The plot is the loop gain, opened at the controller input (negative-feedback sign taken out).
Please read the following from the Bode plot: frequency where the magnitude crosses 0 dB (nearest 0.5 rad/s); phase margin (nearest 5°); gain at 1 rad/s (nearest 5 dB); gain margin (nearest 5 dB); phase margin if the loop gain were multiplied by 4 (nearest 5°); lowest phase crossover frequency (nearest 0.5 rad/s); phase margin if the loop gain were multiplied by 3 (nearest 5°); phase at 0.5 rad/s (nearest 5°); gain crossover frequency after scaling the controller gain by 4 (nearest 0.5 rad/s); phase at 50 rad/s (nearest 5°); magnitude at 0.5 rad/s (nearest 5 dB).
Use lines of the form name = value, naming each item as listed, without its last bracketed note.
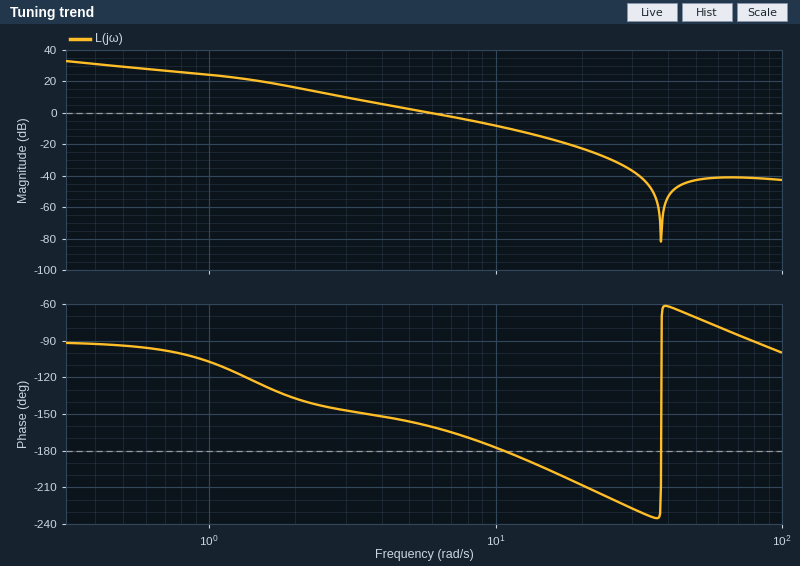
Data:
frequency where the magnitude crosses 0 dB = 6.0 rad/s
phase margin = 20°
gain at 1 rad/s = 25 dB
gain margin = 10 dB
phase margin if the loop gain were multiplied by 4 = -5°
lowest phase crossover frequency = 10.5 rad/s
phase margin if the loop gain were multiplied by 3 = 0°
phase at 0.5 rad/s = -95°
gain crossover frequency after scaling the controller gain by 4 = 12.5 rad/s
phase at 50 rad/s = -70°
magnitude at 0.5 rad/s = 30 dB
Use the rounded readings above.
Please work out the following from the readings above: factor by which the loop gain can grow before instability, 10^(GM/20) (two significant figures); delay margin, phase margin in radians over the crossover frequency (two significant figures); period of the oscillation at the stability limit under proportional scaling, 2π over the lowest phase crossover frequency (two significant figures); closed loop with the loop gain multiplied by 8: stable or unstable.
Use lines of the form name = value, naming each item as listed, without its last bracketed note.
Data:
factor by which the loop gain can grow before instability, 10^(GM/20) = 3.2
delay margin, phase margin in radians over the crossover frequency = 0.058 s
period of the oscillation at the stability limit under proportional scaling, 2π over the lowest phase crossover frequency = 0.60 s
closed loop with the loop gain multiplied by 8: stable or unstable = unstable
